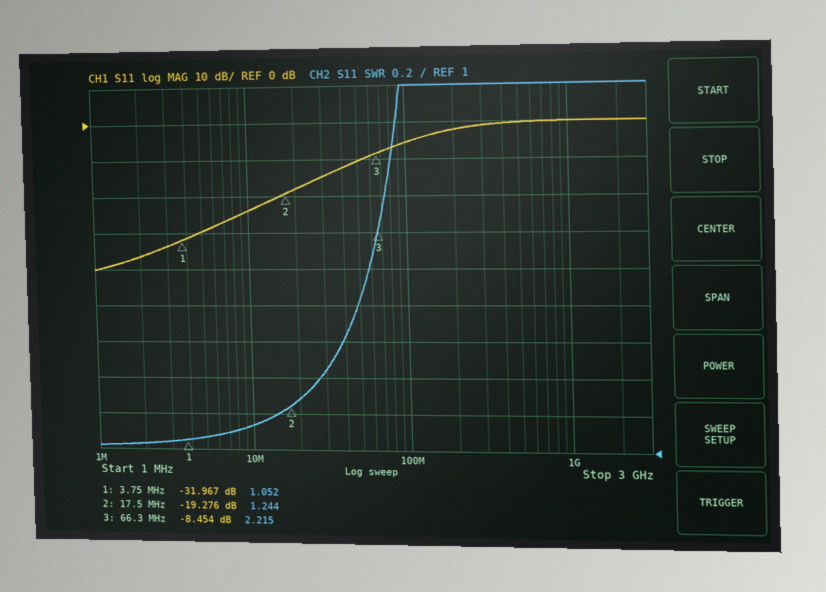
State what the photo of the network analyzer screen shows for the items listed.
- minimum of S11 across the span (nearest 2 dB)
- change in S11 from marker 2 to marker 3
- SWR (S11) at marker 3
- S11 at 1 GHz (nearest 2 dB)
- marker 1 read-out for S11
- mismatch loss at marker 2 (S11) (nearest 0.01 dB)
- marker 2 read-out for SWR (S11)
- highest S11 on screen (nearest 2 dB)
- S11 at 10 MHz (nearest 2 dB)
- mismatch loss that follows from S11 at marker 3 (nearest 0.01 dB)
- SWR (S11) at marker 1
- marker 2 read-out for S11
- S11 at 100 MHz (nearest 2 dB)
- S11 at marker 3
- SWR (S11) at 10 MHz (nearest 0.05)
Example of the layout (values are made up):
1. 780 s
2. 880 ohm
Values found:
1. -40 dB
2. 10.822 dB
3. 2.215
4. 0 dB
5. -31.967 dB
6. 0.05 dB
7. 1.244
8. 0 dB
9. -24 dB
10. 0.67 dB
11. 1.052
12. -19.276 dB
13. -6 dB
14. -8.454 dB
15. 1.15
